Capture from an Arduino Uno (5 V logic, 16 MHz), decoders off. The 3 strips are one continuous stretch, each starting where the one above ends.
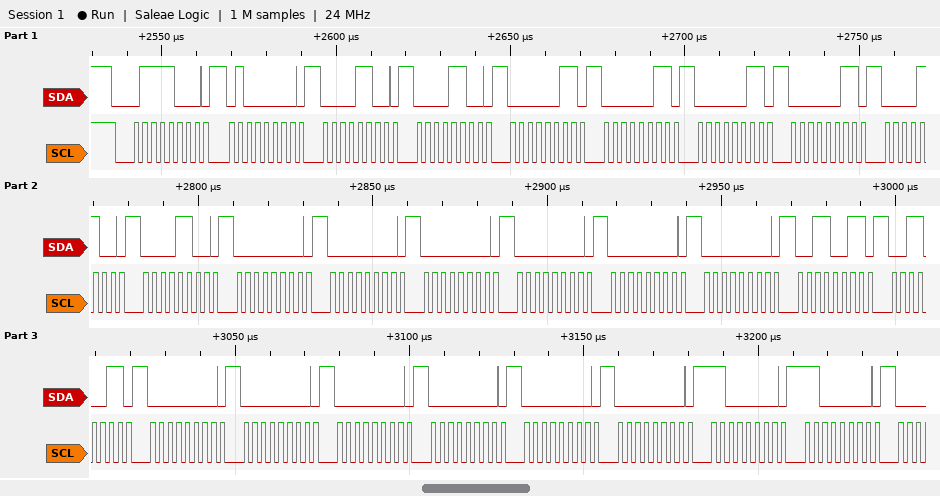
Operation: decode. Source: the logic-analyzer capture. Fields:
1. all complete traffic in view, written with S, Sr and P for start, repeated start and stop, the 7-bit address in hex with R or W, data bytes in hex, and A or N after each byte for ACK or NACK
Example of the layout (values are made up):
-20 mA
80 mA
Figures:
S 3CW A 40 A 0C A 0C A 03 A 03 A 03 A 03 A 0C A 0C A 00 A 00 A 00 A 00 A 00 A 00 A 33 A 33 A 00 A 00 A 00 A 00 A 00 A 00 A C0 A C0 A
